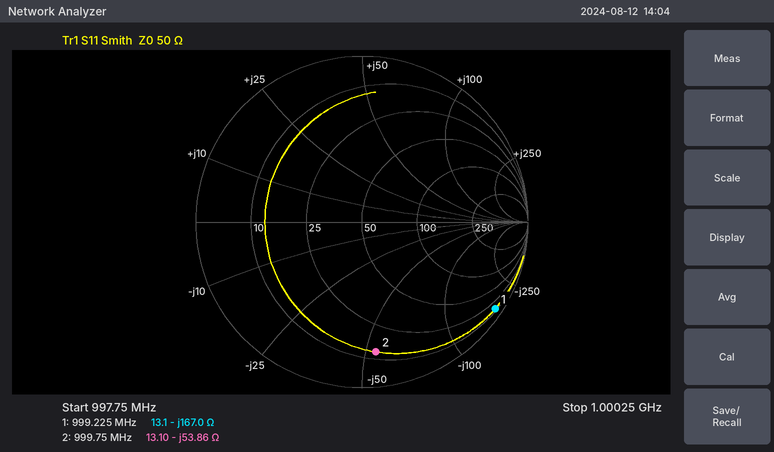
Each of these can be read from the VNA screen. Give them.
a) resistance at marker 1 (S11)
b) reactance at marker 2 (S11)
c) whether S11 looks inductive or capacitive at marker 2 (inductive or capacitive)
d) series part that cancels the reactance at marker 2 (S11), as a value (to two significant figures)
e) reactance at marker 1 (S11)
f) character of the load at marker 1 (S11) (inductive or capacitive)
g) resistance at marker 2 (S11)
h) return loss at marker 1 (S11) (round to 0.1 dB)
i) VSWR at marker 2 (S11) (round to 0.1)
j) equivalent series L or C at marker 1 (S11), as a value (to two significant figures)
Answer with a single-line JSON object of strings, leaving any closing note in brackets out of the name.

{"resistance at marker 1": "13.1 Ω", "reactance at marker 2": "-53.86 Ω", "whether S11 looks inductive or capacitive at marker 2": "capacitive", "series part that cancels the reactance at marker 2 (S11), as a value": "8.6 nH", "reactance at marker 1": "-167.0 Ω", "character of the load at marker 1 (S11)": "capacitive", "resistance at marker 2": "13.10 Ω", "return loss at marker 1 (S11)": "0.4 dB", "VSWR at marker 2 (S11)": "8.4", "equivalent series L or C at marker 1 (S11), as a value": "950 fF"}
